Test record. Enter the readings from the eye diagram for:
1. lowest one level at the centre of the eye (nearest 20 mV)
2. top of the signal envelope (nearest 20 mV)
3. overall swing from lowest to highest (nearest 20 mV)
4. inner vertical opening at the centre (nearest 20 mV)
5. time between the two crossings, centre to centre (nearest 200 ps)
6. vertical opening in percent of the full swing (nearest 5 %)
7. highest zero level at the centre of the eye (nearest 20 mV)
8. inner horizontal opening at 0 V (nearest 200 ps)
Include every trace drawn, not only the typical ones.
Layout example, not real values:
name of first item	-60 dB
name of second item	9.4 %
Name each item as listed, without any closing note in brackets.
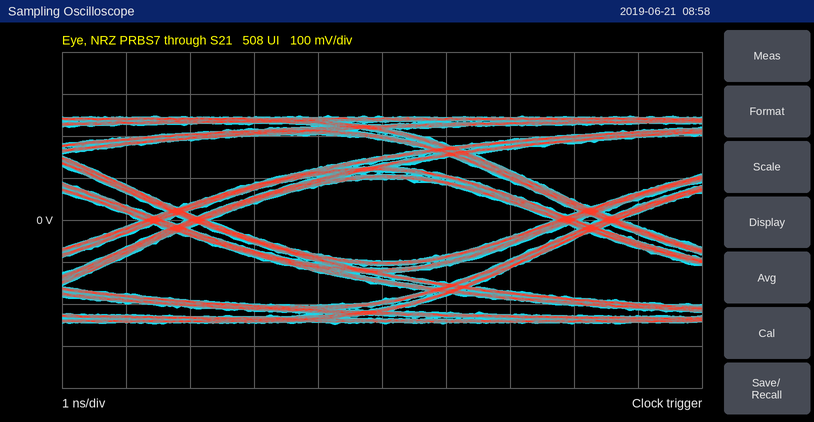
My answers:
lowest one level at the centre of the eye	100 mV
top of the signal envelope	240 mV
overall swing from lowest to highest	500 mV
inner vertical opening at the centre	200 mV
time between the two crossings, centre to centre	6.4 ns
vertical opening in percent of the full swing	40 %
highest zero level at the centre of the eye	-100 mV
inner horizontal opening at 0 V	5.4 ns
